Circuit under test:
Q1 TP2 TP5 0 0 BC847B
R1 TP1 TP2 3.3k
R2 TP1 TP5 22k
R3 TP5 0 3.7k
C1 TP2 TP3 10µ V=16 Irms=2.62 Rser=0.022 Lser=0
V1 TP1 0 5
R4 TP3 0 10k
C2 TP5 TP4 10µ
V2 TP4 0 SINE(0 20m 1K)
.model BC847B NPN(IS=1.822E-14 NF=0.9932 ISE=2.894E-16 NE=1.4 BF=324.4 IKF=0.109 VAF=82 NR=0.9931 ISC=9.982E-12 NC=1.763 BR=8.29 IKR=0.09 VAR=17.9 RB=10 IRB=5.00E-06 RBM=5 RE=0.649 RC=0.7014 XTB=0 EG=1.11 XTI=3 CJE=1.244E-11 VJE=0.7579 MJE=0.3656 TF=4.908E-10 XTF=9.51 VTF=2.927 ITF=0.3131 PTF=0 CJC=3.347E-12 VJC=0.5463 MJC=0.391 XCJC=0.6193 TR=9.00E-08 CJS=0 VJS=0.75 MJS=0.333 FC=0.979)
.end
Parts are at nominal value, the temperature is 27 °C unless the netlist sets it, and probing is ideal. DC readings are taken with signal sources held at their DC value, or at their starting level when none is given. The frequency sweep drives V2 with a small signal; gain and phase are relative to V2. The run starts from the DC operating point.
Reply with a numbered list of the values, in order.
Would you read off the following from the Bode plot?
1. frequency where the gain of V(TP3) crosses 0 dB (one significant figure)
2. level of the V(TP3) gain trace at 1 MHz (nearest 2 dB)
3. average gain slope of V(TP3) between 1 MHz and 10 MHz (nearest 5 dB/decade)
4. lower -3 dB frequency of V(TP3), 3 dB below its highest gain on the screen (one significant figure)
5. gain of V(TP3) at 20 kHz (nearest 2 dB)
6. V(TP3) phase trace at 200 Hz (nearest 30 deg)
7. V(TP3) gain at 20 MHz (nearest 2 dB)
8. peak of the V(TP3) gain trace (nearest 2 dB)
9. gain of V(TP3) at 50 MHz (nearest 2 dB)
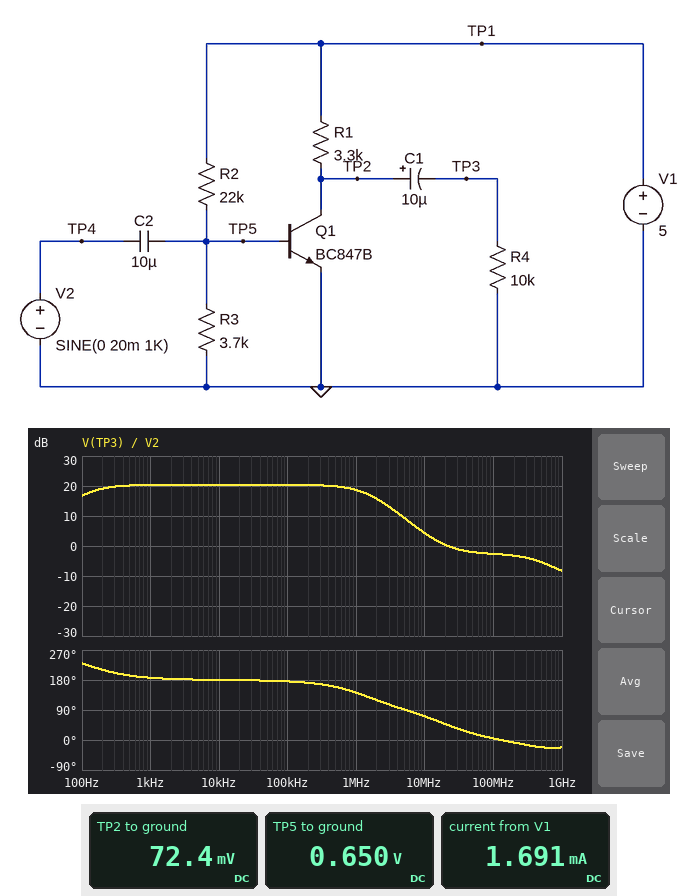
1. 20 MHz
2. 18 dB
3. -15 dB/decade
4. 100 Hz
5. 20 dB
6. 210 deg
7. 0 dB
8. 20 dB
9. -2 dB
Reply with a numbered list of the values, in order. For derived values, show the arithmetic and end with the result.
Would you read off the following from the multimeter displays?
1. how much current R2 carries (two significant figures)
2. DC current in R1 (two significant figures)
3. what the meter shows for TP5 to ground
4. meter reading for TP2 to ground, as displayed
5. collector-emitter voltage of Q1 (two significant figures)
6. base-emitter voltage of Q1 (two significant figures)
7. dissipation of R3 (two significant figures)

1. (5 V - 650 mV) / 22 kΩ = 200 µA
2. (5 V - 72.4 mV) / 3.3 kΩ = 1.5 mA
3. 0.650 V
4. 72.4 mV
5. 72.4 mV = 72 mV
6. 650 mV = 650 mV
7. (650 mV)^2 / 3.7 kΩ = 110 µW
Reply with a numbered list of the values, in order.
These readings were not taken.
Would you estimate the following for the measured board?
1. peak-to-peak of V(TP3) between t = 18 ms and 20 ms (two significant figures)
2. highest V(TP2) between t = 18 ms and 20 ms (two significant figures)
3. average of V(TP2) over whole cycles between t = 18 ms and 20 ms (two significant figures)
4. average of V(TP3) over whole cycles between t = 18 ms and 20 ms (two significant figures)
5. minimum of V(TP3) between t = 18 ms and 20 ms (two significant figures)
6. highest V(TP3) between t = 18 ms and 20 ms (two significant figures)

1. 2.5 V
2. 2.5 V
3. 1.1 V
4. 880 mV
5. -210 mV
6. 2.3 V
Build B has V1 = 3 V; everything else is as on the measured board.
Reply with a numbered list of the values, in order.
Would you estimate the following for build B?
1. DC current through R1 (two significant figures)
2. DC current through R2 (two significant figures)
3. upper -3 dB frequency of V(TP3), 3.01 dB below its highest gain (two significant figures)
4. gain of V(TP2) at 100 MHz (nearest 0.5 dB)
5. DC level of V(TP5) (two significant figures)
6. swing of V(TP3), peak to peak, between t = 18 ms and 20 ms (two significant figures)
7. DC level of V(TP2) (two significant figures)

1. 370 nA
2. 120 µA
3. 1.2 GHz
4. -0.5 dB
5. 430 mV
6. 1.6 mV
7. 3.0 V
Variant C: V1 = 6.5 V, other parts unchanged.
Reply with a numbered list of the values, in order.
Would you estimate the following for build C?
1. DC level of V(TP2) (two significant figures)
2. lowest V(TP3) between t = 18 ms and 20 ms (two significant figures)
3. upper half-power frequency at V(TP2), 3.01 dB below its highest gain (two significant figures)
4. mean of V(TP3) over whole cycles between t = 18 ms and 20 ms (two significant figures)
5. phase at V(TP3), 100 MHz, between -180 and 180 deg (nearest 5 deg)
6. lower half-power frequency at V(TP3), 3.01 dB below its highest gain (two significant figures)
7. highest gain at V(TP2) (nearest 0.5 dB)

1. 43 mV
2. -150 mV
3. 1.3 MHz
4. 630 mV
5. -5 deg
6. 180 Hz
7. 9.0 dB
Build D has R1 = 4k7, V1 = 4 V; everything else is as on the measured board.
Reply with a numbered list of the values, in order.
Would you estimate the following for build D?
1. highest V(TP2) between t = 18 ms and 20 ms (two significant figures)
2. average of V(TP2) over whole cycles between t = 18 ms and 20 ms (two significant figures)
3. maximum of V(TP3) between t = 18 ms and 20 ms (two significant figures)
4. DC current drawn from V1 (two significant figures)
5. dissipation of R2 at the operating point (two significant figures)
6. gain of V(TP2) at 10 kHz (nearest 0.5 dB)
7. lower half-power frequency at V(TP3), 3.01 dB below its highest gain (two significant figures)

1. 3.7 V
2. 3.5 V
3. 170 mV
4. 250 µA
5. 530 µW
6. 21.5 dB
7. 5.4 Hz
